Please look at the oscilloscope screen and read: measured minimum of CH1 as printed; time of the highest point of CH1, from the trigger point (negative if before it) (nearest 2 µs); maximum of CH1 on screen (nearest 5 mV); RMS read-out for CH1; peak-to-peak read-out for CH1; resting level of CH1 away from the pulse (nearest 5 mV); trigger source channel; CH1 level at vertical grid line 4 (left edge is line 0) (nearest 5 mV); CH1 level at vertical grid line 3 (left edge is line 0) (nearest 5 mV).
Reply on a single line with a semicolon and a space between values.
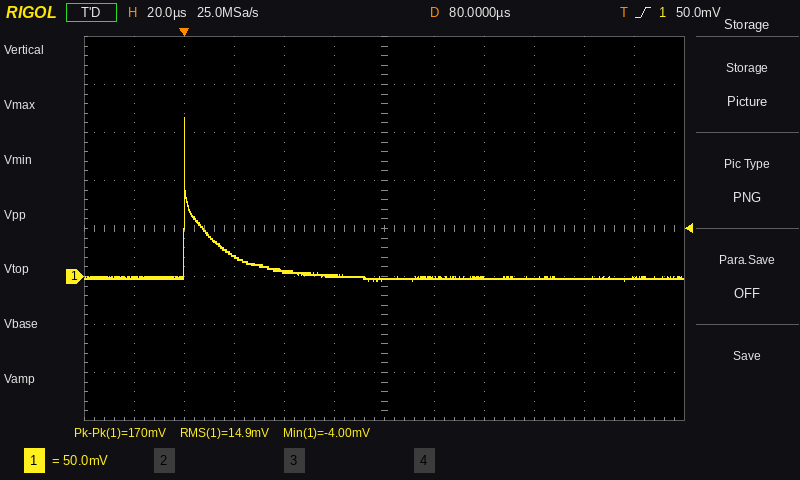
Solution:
-4.00 mV; 0 µs; 165 mV; 14.9 mV; 170 mV; 0 mV; CH1; 5 mV; 20 mV
